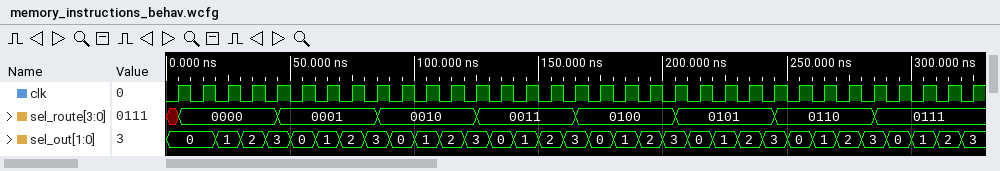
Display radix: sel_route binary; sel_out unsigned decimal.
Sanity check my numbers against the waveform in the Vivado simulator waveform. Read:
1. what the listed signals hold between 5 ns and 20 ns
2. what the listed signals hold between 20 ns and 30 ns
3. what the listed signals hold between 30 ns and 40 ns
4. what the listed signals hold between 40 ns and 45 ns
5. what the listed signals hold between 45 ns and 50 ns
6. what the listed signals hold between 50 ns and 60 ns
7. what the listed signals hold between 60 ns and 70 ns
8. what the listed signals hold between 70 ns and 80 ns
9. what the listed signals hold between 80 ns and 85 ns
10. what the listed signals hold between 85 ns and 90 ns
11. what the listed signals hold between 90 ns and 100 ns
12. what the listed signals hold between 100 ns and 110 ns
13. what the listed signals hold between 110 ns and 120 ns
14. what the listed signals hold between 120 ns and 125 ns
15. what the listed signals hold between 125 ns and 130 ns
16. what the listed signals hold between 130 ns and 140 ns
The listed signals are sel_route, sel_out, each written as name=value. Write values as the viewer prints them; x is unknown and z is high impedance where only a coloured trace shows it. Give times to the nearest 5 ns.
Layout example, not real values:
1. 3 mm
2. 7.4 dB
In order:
1. sel_route=0000, sel_out=0
2. sel_route=0000, sel_out=1
3. sel_route=0000, sel_out=2
4. sel_route=0000, sel_out=3
5. sel_route=0001, sel_out=3
6. sel_route=0001, sel_out=0
7. sel_route=0001, sel_out=1
8. sel_route=0001, sel_out=2
9. sel_route=0001, sel_out=3
10. sel_route=0010, sel_out=3
11. sel_route=0010, sel_out=0
12. sel_route=0010, sel_out=1
13. sel_route=0010, sel_out=2
14. sel_route=0010, sel_out=3
15. sel_route=0011, sel_out=3
16. sel_route=0011, sel_out=0
